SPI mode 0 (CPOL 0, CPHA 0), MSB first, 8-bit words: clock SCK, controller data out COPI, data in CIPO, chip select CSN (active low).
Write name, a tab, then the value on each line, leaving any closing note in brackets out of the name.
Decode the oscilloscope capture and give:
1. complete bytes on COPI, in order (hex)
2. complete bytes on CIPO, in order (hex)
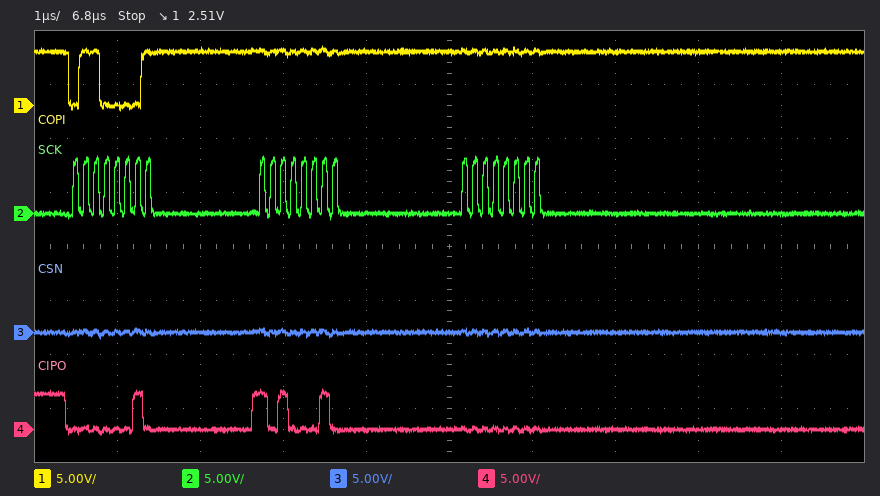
complete bytes on COPI, in order	0x61 0xFF 0xFF
complete bytes on CIPO, in order	0x02 0xA2 0x00
